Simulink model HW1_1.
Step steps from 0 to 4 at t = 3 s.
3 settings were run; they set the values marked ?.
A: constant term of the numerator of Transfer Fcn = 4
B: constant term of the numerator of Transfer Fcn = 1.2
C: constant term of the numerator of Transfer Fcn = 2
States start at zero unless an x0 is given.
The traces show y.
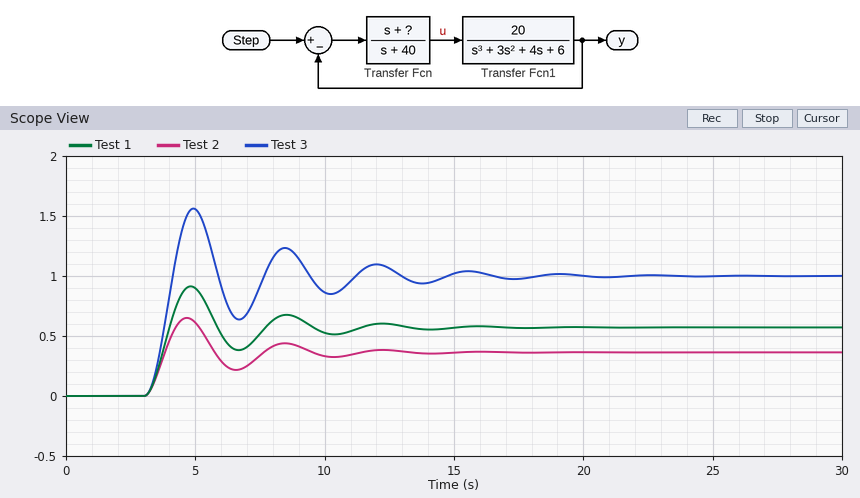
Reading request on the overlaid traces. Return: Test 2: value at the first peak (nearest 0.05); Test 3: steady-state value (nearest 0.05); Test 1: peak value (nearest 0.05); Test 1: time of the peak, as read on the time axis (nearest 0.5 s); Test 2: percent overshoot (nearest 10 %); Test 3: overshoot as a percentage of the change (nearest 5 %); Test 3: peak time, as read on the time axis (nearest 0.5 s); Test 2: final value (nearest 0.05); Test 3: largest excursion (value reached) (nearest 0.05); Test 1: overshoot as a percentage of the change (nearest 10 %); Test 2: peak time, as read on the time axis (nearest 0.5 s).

0.65
1.00
0.90
5.0 s
80 %
55 %
5.0 s
0.35
1.55
60 %
4.5 s
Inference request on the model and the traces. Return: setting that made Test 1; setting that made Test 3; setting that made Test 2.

C
A
B
